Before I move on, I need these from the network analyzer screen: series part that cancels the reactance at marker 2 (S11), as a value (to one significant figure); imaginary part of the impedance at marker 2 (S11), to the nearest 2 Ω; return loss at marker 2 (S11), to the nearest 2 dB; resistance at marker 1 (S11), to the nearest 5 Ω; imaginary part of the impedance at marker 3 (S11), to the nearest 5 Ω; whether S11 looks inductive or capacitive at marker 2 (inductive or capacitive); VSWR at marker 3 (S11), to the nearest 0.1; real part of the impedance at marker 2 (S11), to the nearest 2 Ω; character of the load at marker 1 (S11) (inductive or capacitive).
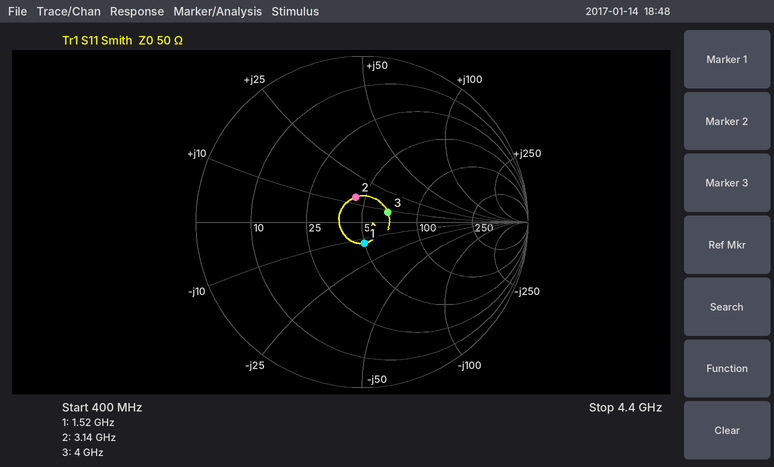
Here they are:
4 pF
+14 Ω
16 dB
50 Ω
+10 Ω
inductive
1.4
44 Ω
capacitive
